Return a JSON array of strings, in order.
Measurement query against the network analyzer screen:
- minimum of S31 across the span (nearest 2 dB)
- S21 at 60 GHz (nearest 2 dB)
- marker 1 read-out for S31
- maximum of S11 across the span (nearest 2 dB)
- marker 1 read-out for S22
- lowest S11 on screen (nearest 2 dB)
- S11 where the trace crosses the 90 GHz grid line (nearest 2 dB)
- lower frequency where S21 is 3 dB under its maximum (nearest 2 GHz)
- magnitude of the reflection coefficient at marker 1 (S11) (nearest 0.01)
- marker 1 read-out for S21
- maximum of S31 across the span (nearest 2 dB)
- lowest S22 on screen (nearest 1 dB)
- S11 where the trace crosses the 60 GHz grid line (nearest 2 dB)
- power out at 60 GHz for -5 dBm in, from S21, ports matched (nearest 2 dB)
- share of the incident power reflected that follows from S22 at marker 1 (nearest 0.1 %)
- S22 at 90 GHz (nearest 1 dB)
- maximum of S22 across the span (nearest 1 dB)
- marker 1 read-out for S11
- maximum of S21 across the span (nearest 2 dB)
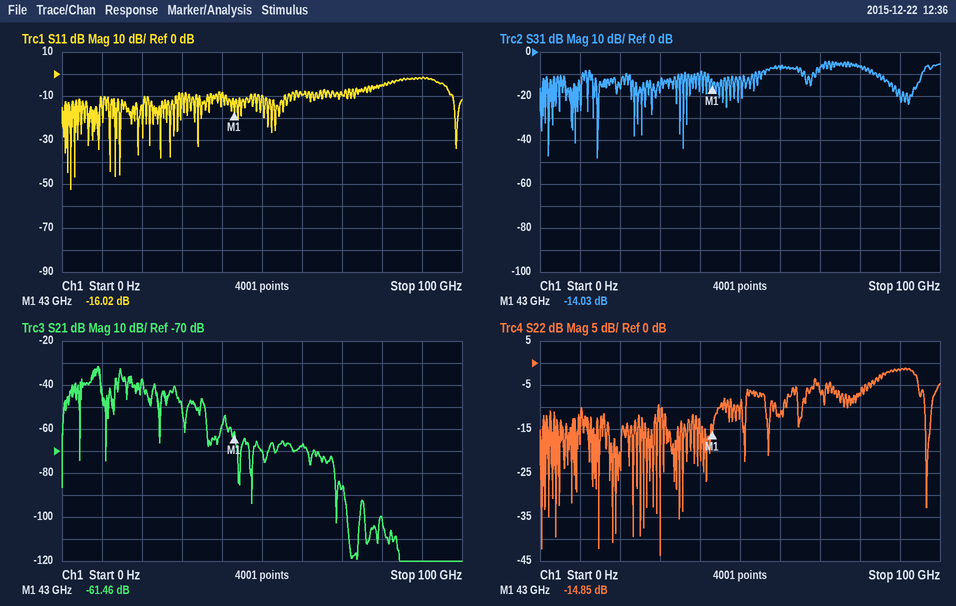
["-48 dB", "-68 dB", "-14.03 dB", "-2 dB", "-14.85 dB", "-52 dB", "-2 dB", "8 GHz", "0.16", "-61.46 dB", "-4 dB", "-44 dB", "-10 dB", "-72 dBm", "3.3 %", "-2 dB", "-1 dB", "-16.02 dB", "-32 dB"]
